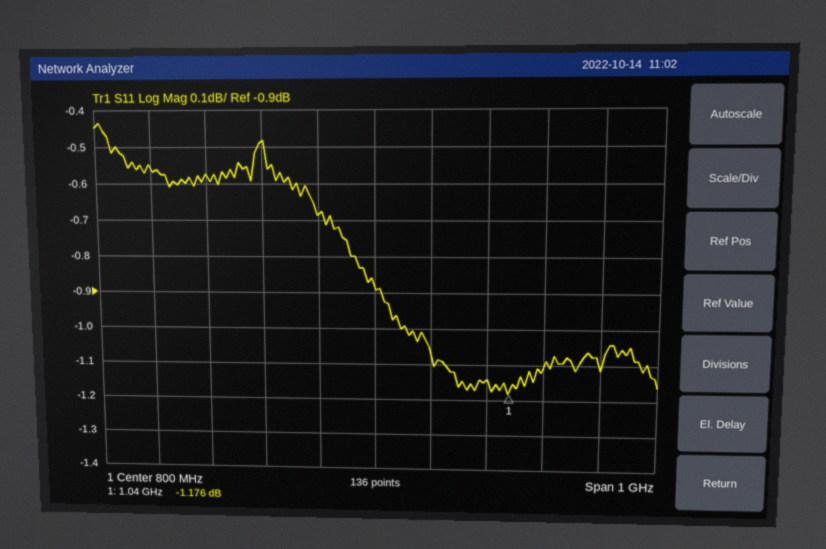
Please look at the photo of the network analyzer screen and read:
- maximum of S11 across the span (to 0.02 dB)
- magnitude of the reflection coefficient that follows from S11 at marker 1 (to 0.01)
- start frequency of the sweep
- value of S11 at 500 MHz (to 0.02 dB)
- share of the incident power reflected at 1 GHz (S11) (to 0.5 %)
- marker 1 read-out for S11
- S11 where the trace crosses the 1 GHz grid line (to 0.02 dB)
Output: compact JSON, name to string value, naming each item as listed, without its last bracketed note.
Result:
{"maximum of S11 across the span": "-0.44 dB", "magnitude of the reflection coefficient that follows from S11 at marker 1": "0.87", "start frequency of the sweep": "300 MHz", "value of S11 at 500 MHz": "-0.58 dB", "share of the incident power reflected at 1 GHz (S11)": "77.0 %", "marker 1 read-out for S11": "-1.176 dB", "S11 where the trace crosses the 1 GHz grid line": "-1.14 dB"}
